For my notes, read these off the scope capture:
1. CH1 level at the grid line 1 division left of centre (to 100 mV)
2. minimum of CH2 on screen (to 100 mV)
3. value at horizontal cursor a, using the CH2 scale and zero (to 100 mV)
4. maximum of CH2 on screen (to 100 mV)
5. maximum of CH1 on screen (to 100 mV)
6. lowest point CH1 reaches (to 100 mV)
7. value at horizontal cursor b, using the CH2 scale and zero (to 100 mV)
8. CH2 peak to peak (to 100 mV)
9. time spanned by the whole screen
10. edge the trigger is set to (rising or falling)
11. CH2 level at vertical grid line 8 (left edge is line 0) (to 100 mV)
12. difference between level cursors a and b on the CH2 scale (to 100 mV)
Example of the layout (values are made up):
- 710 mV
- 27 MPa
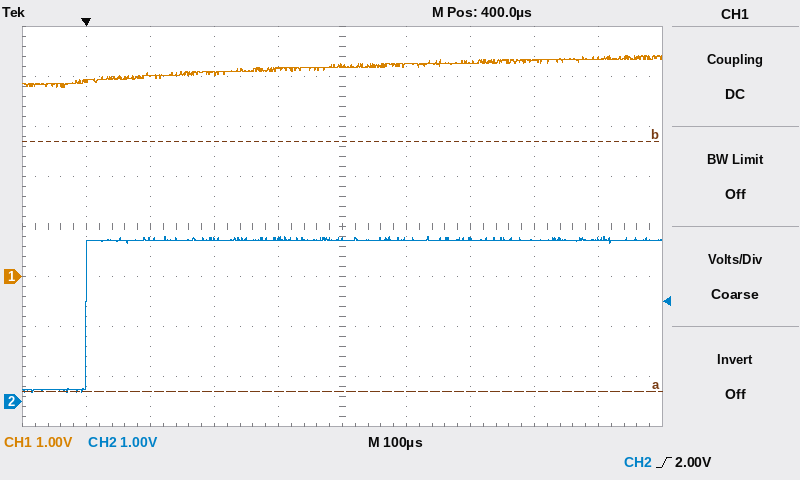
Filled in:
- 4.1 V
- 200 mV
- 200 mV
- 3.3 V
- 4.4 V
- 3.8 V
- 5.2 V
- 3.1 V
- 1 ms
- rising
- 3.2 V
- 5.0 V
